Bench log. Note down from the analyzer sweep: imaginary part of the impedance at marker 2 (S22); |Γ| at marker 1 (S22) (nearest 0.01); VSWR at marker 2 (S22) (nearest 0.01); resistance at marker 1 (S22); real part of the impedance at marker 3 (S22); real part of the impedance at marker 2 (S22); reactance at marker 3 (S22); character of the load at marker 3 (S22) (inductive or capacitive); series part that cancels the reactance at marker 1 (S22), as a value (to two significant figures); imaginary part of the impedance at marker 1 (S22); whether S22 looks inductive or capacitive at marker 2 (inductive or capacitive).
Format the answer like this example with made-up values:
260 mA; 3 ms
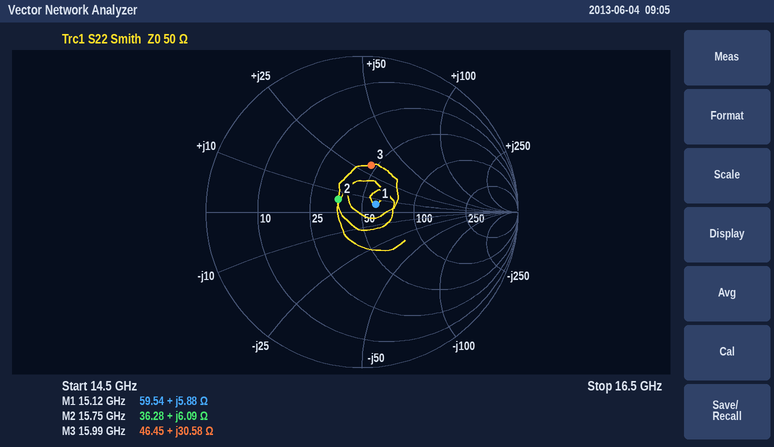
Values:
+6.09 Ω; 0.10; 1.42; 59.54 Ω; 46.45 Ω; 36.28 Ω; +30.58 Ω; inductive; 1.8 pF; +5.88 Ω; inductive
